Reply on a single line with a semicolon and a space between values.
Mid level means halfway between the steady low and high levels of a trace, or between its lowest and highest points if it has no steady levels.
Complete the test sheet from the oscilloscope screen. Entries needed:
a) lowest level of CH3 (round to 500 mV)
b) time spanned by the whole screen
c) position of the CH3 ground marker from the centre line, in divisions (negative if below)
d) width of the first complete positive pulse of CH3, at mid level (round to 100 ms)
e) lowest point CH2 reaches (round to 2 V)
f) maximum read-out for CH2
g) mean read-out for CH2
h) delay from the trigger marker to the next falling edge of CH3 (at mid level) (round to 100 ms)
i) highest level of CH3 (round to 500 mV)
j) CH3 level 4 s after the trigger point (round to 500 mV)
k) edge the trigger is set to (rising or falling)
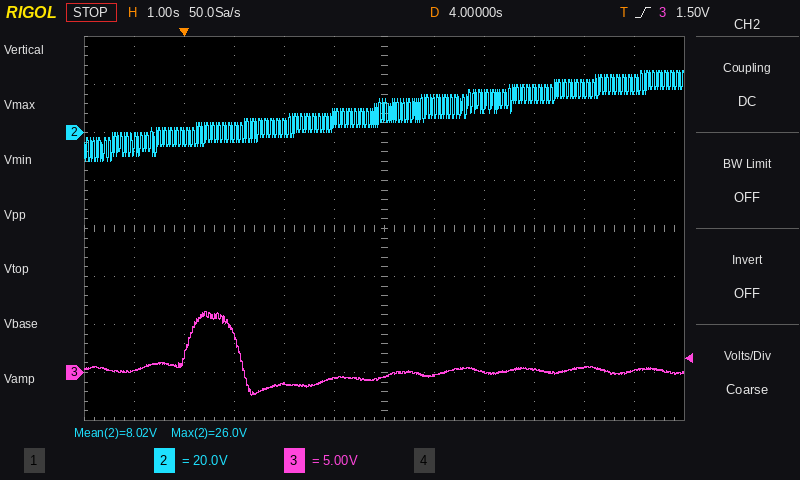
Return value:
-2.5 V; 12 s; -3.0 div; 1.1 s; -12 V; 26.0 V; 8.02 V; 1.1 s; 6.5 V; -500 mV; rising
